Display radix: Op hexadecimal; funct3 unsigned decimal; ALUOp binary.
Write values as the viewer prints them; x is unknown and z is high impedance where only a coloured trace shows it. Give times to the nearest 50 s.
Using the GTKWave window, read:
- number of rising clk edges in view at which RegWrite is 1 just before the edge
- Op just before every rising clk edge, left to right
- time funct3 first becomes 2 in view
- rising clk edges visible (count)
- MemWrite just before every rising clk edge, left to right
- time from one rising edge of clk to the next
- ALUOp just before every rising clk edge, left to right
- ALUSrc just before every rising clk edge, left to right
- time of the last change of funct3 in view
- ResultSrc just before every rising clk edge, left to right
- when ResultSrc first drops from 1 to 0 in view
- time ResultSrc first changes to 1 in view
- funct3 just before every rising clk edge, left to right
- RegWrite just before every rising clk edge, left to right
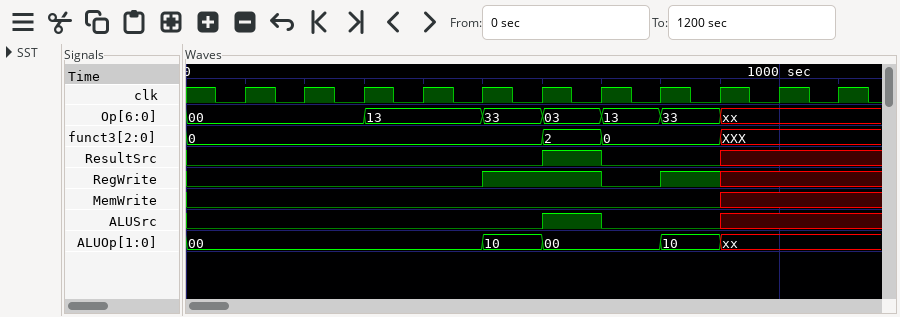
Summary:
3
00, 00, 00, 13, 13, 33, 03, 13, 33, xx, xx
600 s
11
0 0 0 0 0 0 0 0 0 x x
100 s
00, 00, 00, 00, 00, 10, 00, 00, 10, xx, xx
0 0 0 0 0 0 1 0 0 x x
900 s
0 0 0 0 0 0 1 0 0 x x
700 s
600 s
0, 0, 0, 0, 0, 0, 2, 0, 0, XXX, XXX
0 0 0 0 0 1 1 0 1 x x
